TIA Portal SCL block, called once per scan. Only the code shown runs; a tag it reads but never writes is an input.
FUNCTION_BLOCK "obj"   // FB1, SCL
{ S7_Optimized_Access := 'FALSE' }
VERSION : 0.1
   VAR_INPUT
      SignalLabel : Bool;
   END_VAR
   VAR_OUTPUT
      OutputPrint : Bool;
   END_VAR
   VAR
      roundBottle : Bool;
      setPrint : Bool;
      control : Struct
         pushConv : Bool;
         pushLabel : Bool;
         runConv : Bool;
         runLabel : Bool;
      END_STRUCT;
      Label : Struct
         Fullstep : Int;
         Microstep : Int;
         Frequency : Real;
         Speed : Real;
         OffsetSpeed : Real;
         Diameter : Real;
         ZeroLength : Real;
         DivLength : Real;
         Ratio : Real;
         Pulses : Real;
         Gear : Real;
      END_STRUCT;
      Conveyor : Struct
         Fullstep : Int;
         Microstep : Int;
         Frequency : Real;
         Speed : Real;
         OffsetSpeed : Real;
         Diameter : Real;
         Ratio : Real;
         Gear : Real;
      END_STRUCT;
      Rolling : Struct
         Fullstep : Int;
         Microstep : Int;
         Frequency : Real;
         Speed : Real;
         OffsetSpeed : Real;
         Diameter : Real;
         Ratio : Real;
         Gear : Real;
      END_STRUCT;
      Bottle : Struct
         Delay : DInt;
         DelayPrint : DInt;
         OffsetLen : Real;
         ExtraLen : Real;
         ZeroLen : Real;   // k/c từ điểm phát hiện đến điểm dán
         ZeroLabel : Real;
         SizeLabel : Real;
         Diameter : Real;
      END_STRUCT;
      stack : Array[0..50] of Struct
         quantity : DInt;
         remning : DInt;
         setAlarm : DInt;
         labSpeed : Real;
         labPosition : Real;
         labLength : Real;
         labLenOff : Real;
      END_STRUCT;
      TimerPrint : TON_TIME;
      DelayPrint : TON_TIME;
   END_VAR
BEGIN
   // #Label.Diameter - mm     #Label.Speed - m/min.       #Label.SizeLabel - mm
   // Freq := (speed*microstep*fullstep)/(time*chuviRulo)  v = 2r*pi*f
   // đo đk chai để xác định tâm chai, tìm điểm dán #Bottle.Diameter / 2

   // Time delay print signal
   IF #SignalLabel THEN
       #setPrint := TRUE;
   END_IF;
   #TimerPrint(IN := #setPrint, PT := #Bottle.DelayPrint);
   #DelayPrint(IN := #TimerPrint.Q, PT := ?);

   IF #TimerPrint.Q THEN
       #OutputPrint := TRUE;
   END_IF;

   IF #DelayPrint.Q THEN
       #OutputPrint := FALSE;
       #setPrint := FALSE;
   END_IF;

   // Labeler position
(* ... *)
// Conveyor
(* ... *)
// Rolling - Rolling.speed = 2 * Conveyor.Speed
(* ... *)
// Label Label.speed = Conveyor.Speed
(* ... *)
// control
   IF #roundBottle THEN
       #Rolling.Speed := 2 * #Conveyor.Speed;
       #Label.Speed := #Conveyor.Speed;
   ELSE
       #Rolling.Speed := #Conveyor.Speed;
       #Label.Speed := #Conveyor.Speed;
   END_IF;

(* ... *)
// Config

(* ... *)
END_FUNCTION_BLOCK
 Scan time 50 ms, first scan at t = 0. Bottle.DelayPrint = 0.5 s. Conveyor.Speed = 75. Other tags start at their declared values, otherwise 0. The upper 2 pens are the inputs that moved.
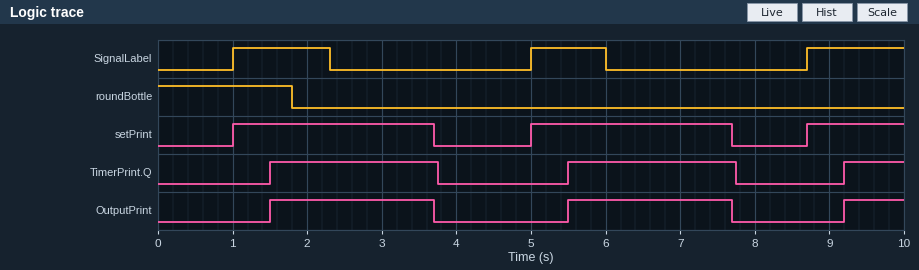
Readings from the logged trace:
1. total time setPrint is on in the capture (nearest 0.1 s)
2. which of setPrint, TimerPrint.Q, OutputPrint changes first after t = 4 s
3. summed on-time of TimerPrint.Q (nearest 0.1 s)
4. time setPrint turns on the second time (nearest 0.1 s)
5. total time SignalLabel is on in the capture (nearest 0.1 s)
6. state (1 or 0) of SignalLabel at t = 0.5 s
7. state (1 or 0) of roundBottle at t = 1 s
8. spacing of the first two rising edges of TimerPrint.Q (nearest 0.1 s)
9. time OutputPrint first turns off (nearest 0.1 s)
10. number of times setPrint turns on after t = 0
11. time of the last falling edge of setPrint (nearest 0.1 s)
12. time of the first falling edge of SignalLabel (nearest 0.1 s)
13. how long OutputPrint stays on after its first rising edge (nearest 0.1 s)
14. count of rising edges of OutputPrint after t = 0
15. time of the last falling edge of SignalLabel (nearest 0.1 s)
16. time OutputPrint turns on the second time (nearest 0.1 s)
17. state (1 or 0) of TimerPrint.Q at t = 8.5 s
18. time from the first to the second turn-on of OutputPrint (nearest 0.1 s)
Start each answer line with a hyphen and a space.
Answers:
- 6.7 s
- setPrint
- 5.3 s
- 5.0 s
- 3.6 s
- 0
- 1
- 4.0 s
- 3.7 s
- 3
- 7.7 s
- 2.3 s
- 2.2 s
- 3
- 6.0 s
- 5.5 s
- 0
- 4.0 s
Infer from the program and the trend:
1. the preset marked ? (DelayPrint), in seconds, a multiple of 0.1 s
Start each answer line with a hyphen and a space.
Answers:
- 2.2 s
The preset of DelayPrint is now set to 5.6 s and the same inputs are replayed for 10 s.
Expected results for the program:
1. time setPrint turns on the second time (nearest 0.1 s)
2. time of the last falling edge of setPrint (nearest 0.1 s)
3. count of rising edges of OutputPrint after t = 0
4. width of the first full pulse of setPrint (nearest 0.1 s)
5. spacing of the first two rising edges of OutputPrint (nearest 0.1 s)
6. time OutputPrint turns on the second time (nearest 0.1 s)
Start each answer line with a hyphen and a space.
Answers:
- 8.7 s
- 7.1 s
- 2
- 6.1 s
- 7.7 s
- 9.2 s
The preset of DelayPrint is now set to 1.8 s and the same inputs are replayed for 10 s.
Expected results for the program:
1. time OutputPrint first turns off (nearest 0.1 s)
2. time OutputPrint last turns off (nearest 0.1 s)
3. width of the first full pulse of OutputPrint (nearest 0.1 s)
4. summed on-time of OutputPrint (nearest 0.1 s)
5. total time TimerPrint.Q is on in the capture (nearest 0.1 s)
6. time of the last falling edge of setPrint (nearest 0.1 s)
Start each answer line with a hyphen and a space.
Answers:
- 3.3 s
- 7.3 s
- 1.8 s
- 4.4 s
- 4.5 s
- 7.3 s
